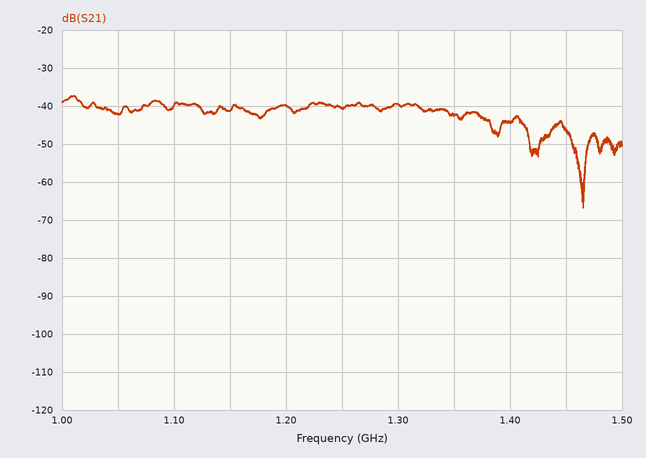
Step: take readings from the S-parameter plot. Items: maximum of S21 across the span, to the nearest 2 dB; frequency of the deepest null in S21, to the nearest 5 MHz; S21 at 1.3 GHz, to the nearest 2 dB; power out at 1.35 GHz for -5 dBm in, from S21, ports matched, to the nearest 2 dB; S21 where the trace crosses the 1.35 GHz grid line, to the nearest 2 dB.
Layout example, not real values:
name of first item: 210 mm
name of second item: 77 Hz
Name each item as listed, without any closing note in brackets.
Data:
maximum of S21 across the span, to the nearest 2 dB: -38 dB
frequency of the deepest null in S21, to the nearest 5 MHz: 1.465 GHz
S21 at 1.3 GHz, to the nearest 2 dB: -40 dB
power out at 1.35 GHz for -5 dBm in, from S21, ports matched, to the nearest 2 dB: -48 dBm
S21 where the trace crosses the 1.35 GHz grid line, to the nearest 2 dB: -42 dB
